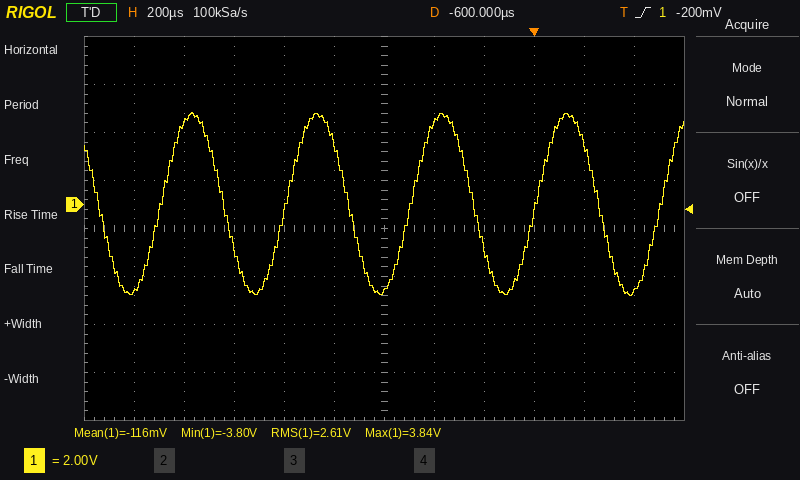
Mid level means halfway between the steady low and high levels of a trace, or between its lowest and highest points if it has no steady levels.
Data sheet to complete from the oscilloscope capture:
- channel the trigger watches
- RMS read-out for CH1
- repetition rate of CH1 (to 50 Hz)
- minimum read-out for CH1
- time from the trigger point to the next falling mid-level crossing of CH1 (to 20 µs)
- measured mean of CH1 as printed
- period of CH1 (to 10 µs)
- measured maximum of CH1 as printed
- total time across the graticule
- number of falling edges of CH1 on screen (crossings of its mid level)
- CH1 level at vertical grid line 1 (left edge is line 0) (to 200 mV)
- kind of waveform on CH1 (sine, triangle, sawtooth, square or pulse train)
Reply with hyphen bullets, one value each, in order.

- CH1
- 2.61 V
- 2.00 kHz
- -3.80 V
- 260 µs
- -116 mV
- 500 µs
- 3.84 V
- 2.4 ms
- 5
- -3.6 V
- sine
